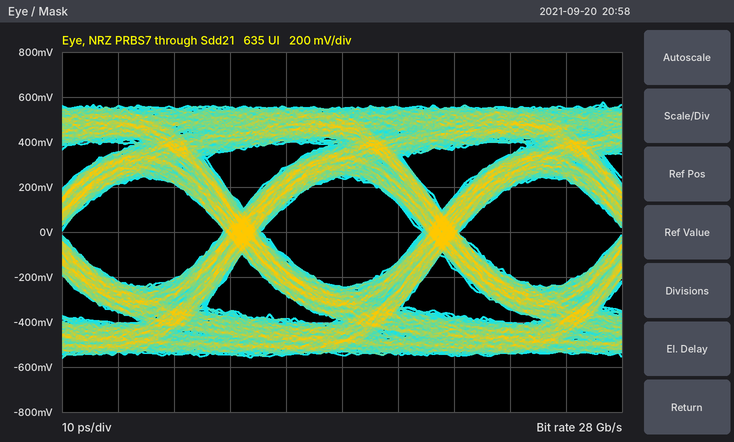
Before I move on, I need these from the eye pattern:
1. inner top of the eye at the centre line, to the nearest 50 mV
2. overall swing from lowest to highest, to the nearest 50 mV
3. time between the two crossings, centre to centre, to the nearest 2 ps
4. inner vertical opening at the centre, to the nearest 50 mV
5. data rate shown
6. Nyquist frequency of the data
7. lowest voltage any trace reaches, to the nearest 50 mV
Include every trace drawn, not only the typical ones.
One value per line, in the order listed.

250 mV
1.15 V
36 ps
500 mV
28 Gb/s
14 GHz
-550 mV
